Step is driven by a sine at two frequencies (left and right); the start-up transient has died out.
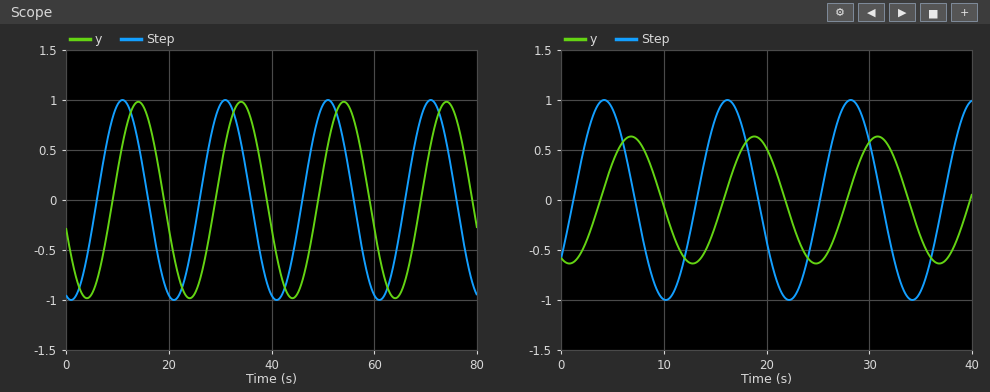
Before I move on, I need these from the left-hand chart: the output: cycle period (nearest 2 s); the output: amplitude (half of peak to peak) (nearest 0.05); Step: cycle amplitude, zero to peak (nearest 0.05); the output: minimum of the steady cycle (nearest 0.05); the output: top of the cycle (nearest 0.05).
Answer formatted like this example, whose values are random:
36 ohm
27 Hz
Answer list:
20 s
1.00
1.00
-1.00
1.00
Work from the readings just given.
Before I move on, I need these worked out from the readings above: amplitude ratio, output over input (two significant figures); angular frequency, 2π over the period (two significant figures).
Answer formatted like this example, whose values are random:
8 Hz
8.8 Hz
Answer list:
1.0
0.31 rad/s
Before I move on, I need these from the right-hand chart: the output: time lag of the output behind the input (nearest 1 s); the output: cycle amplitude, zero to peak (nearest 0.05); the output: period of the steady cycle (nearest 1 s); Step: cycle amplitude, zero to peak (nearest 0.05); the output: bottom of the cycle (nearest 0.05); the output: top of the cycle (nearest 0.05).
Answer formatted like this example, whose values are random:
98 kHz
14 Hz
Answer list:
3 s
0.65
12 s
1.00
-0.65
0.65
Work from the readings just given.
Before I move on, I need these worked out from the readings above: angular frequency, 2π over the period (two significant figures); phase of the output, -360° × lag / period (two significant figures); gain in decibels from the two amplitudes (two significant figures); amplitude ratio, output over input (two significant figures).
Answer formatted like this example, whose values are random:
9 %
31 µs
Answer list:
0.52 rad/s
-90°
-3.7 dB
0.65
